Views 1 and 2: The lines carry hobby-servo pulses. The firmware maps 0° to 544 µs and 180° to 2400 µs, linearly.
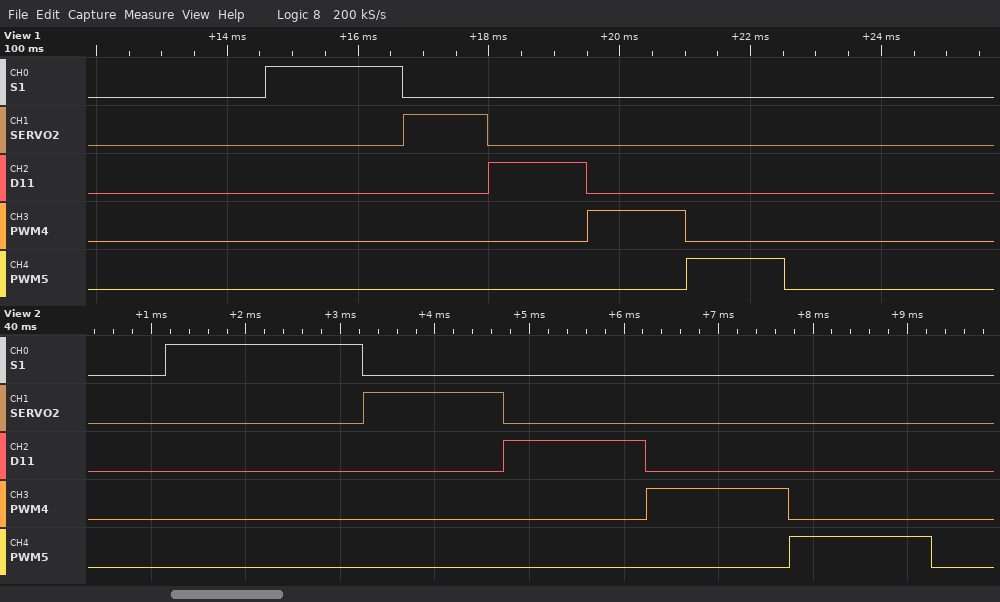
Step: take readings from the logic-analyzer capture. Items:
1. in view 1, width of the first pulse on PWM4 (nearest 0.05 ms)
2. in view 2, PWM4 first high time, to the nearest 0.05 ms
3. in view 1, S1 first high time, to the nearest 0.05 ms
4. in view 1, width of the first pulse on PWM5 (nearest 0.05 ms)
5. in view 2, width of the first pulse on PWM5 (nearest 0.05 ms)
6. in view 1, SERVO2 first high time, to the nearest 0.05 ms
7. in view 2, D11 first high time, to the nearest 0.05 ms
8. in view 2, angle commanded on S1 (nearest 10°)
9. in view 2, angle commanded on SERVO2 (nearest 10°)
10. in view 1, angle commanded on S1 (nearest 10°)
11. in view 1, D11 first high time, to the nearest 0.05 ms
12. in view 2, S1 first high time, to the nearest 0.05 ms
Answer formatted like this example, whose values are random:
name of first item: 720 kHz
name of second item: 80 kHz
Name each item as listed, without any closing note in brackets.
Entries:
in view 1, width of the first pulse on PWM4: 1.50 ms
in view 2, PWM4 first high time, to the nearest 0.05 ms: 1.50 ms
in view 1, S1 first high time, to the nearest 0.05 ms: 2.10 ms
in view 1, width of the first pulse on PWM5: 1.50 ms
in view 2, width of the first pulse on PWM5: 1.50 ms
in view 1, SERVO2 first high time, to the nearest 0.05 ms: 1.30 ms
in view 2, D11 first high time, to the nearest 0.05 ms: 1.50 ms
in view 2, angle commanded on S1: 150°
in view 2, angle commanded on SERVO2: 90°
in view 1, angle commanded on S1: 150°
in view 1, D11 first high time, to the nearest 0.05 ms: 1.50 ms
in view 2, S1 first high time, to the nearest 0.05 ms: 2.10 ms
